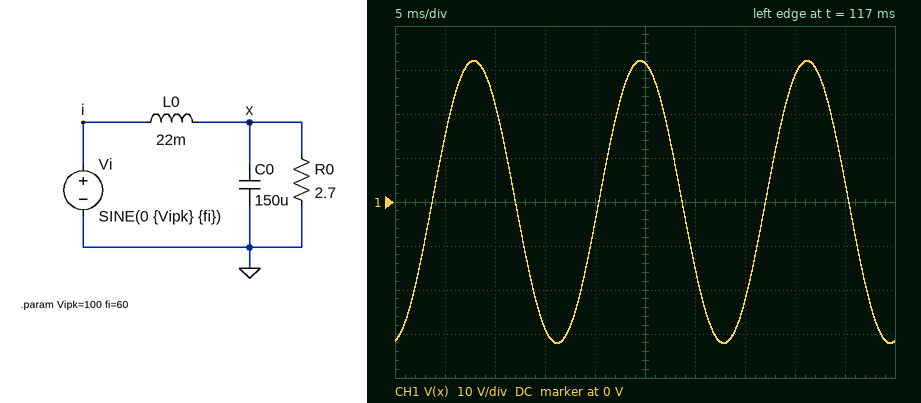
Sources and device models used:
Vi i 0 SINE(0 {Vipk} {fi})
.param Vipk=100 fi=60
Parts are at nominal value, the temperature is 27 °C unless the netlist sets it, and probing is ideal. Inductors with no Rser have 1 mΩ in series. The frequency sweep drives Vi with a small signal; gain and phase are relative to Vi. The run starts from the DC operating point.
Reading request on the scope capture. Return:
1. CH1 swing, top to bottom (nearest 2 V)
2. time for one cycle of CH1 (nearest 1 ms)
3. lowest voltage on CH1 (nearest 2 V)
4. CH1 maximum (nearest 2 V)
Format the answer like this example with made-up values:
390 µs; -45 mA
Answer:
64 V; 17 ms; -32 V; 32 V
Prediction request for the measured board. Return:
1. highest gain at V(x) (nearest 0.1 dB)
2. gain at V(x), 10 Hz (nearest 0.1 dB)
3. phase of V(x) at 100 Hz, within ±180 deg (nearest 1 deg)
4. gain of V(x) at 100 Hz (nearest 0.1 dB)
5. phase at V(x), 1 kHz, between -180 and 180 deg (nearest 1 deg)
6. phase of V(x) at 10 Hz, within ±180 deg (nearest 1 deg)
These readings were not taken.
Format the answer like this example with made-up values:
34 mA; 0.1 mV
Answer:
0 dB; -0.9 dB; -93 deg; -14.2 dB; -158 deg; -27 deg
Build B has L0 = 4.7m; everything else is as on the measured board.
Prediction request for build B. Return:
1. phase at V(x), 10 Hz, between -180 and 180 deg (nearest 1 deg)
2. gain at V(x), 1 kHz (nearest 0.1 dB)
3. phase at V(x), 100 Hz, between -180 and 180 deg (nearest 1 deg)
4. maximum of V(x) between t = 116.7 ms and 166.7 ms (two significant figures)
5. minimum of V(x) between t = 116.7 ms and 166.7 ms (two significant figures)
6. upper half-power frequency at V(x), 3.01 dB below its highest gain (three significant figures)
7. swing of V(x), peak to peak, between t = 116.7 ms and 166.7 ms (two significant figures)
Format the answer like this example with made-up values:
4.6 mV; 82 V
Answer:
-6 deg; -29.2 dB; -57 deg; 90 V; -90 V; 116 Hz; 180 V
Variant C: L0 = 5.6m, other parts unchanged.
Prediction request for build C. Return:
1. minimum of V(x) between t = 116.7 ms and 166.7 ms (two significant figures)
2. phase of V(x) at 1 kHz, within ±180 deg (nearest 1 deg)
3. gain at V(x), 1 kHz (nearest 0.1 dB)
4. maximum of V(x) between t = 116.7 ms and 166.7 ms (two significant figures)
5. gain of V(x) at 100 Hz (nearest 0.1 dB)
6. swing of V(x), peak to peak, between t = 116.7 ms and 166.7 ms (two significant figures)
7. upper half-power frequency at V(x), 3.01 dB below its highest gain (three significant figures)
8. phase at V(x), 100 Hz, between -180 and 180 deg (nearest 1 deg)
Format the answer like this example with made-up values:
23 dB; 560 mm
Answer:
-85 V; -158 deg; -30.8 dB; 85 V; -3.3 dB; 170 V; 94.0 Hz; -63 deg
